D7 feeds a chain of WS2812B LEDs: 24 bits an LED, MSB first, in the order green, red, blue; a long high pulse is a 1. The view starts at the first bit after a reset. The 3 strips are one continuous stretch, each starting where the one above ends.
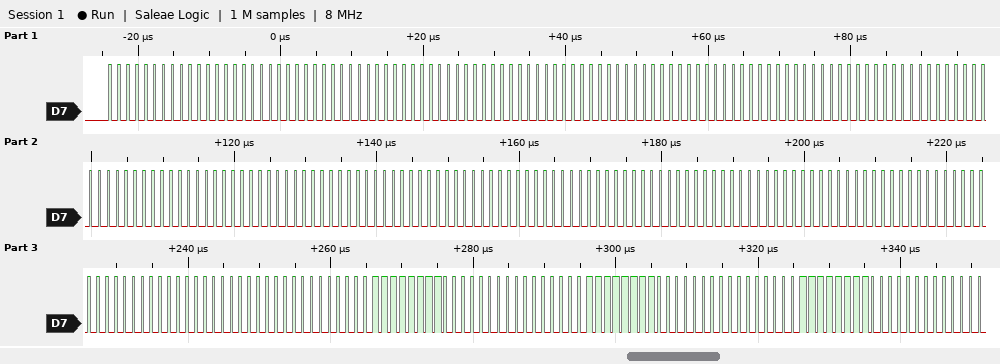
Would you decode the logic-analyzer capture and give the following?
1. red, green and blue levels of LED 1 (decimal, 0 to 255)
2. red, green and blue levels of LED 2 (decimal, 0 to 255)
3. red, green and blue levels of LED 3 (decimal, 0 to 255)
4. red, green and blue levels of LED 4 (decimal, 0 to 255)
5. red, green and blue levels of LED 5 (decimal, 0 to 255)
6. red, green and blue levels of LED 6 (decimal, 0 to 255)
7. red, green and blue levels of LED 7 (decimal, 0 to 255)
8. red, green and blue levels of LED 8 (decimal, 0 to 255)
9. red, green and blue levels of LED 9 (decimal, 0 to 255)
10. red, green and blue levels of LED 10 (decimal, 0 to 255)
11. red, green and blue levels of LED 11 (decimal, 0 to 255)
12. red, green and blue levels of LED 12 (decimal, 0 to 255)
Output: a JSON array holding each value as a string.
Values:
["0, 0, 0", "0, 0, 0", "0, 0, 0", "0, 0, 0", "0, 0, 0", "0, 0, 0", "0, 0, 0", "0, 0, 0", "0, 0, 0", "0, 0, 255", "0, 0, 255", "0, 0, 255"]
